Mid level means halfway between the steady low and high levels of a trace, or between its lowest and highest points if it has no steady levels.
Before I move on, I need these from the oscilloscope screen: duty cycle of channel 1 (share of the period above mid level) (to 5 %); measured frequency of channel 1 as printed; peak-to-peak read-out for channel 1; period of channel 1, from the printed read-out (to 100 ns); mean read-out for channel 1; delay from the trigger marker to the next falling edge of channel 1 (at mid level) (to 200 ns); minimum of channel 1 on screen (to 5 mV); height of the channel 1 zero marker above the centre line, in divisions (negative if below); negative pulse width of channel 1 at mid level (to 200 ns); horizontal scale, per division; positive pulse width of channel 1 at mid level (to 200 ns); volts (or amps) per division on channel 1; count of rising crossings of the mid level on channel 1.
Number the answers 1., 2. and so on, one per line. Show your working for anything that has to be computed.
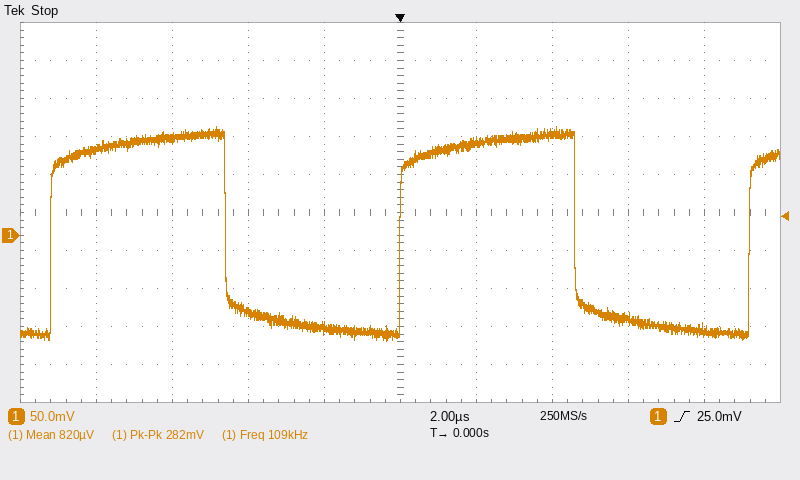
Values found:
1. 50 %
2. 109 kHz
3. 282 mV
4. 1 / 109 kHz ≈ 9.2 µs
5. 820 µV
6. 4.6 µs
7. -140 mV
8. -0.6 div
9. 4.6 µs
10. 2 µs
11. 4.6 µs
12. 50 mV
13. 3
